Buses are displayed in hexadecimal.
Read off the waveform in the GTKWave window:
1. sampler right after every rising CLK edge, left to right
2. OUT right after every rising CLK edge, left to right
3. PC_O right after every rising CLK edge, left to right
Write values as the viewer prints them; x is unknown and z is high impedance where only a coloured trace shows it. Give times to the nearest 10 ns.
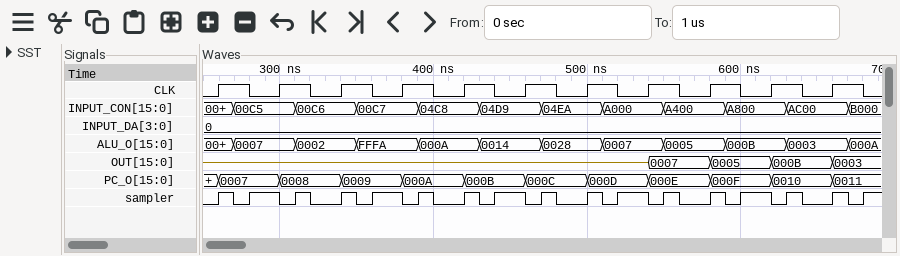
1 0 1 0 1 0 1 0 1 0 1
z, z, z, z, z, z, z, 0007, 0005, 000B, 0003
0007, 0008, 0009, 000A, 000B, 000C, 000D, 000E, 000F, 0010, 0011
